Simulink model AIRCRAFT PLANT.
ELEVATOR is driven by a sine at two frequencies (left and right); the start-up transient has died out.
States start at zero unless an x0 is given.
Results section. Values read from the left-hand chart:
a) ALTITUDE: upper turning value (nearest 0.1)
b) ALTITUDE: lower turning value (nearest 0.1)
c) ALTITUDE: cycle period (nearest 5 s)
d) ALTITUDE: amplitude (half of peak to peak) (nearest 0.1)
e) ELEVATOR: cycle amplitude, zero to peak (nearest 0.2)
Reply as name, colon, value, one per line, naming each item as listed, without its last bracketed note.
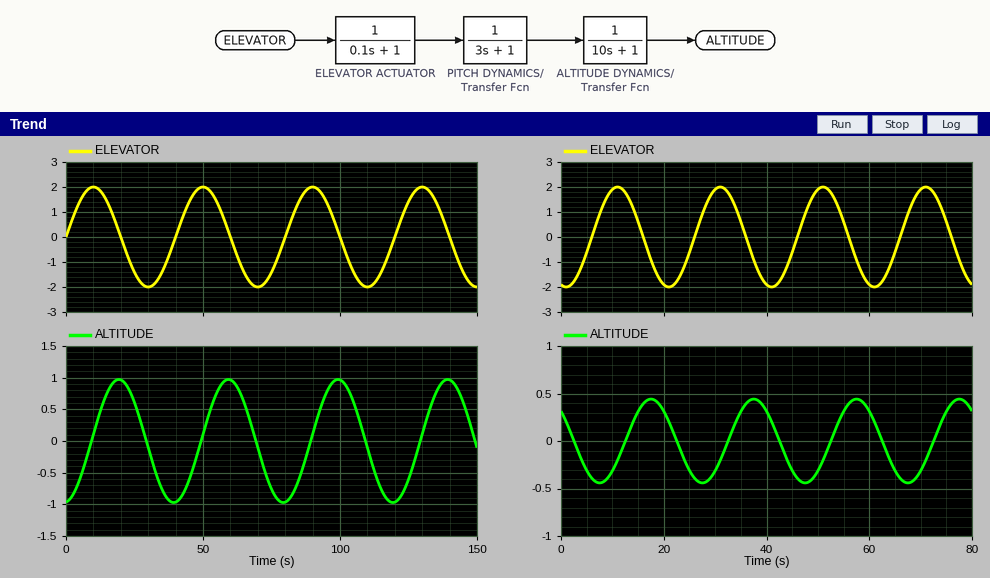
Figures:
ALTITUDE: upper turning value: 1.0
ALTITUDE: lower turning value: -1.0
ALTITUDE: cycle period: 40 s
ALTITUDE: amplitude (half of peak to peak): 1.0
ELEVATOR: cycle amplitude, zero to peak: 2.0
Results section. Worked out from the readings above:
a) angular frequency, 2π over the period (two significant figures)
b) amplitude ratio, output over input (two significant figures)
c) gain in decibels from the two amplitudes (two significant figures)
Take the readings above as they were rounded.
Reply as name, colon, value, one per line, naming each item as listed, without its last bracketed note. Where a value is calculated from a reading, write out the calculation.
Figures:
angular frequency, 2π over the period: 2π / 40 = 0.16 rad/s
amplitude ratio, output over input: 1 / 2 = 0.50
gain in decibels from the two amplitudes: 20 log10(1 / 2) = -6.0 dB
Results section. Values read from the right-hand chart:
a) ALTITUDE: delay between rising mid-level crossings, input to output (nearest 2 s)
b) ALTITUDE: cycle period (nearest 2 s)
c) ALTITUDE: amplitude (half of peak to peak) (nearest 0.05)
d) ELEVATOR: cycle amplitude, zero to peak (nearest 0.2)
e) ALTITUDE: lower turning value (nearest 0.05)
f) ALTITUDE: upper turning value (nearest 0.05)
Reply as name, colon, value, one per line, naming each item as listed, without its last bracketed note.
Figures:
ALTITUDE: delay between rising mid-level crossings, input to output: 6 s
ALTITUDE: cycle period: 20 s
ALTITUDE: amplitude (half of peak to peak): 0.45
ELEVATOR: cycle amplitude, zero to peak: 2.0
ALTITUDE: lower turning value: -0.45
ALTITUDE: upper turning value: 0.45
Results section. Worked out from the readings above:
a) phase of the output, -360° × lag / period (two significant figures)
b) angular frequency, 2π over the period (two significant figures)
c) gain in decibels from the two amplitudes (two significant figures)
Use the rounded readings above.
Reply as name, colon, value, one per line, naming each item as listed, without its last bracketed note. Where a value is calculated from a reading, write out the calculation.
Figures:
phase of the output, -360° × lag / period: -360 × 6 / 20 = -110°
angular frequency, 2π over the period: 2π / 20 = 0.31 rad/s
gain in decibels from the two amplitudes: 20 log10(0.45 / 2) = -13 dB
